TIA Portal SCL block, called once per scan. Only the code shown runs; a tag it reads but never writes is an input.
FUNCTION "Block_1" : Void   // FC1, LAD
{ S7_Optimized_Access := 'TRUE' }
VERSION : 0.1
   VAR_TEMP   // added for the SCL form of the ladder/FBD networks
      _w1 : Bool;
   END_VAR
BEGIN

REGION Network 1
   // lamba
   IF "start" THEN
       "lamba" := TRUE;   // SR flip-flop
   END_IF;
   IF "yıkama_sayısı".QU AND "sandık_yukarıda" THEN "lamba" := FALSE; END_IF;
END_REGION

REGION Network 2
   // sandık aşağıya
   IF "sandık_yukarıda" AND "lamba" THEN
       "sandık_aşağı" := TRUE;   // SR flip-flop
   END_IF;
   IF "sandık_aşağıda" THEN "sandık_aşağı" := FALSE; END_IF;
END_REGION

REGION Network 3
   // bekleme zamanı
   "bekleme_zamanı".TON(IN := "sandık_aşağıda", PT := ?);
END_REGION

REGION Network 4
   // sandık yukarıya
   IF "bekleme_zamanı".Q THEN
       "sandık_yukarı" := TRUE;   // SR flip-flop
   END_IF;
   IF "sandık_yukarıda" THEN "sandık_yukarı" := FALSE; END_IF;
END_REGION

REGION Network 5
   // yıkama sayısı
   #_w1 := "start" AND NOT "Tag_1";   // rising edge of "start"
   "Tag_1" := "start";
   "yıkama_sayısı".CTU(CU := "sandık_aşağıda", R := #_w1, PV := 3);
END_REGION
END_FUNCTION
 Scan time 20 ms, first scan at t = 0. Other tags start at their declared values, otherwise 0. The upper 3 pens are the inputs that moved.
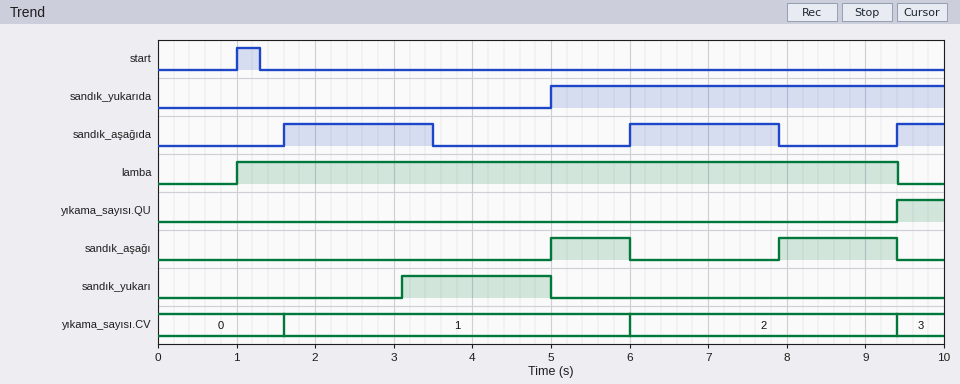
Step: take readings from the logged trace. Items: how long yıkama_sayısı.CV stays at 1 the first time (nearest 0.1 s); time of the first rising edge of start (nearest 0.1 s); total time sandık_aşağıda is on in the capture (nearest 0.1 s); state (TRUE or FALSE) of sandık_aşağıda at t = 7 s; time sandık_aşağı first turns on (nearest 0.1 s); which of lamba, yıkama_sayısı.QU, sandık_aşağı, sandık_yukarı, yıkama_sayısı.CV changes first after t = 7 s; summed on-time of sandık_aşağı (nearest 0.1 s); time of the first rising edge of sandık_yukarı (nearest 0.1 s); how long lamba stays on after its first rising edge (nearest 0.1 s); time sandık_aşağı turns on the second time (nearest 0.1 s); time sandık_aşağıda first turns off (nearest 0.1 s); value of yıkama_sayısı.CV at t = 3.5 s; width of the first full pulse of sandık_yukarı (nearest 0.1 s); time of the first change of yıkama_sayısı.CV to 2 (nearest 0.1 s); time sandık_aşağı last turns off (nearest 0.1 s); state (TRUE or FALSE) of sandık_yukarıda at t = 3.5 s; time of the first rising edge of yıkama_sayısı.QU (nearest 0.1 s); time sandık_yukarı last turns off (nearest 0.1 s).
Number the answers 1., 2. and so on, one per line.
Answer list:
1. 4.4 s
2. 1.0 s
3. 4.4 s
4. TRUE
5. 5.0 s
6. sandık_aşağı
7. 2.5 s
8. 3.1 s
9. 8.4 s
10. 7.9 s
11. 3.5 s
12. 1
13. 1.9 s
14. 6.0 s
15. 9.4 s
16. FALSE
17. 9.4 s
18. 5.0 s
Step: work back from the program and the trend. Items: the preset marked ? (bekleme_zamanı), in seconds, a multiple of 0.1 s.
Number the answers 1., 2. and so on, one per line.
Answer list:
1. 1.5 s
